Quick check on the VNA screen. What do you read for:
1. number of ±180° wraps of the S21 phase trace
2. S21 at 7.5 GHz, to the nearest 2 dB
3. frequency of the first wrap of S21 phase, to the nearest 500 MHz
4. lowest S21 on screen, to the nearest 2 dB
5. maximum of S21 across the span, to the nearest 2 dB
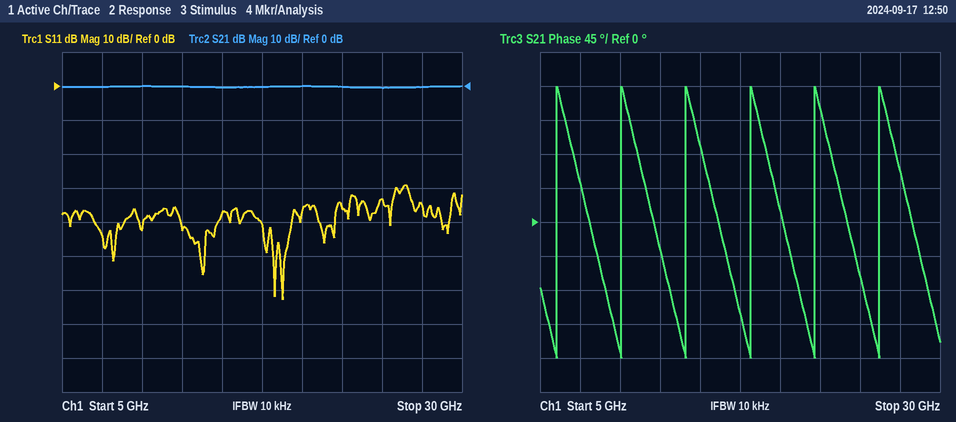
6
0 dB
6.0 GHz
0 dB
0 dB
